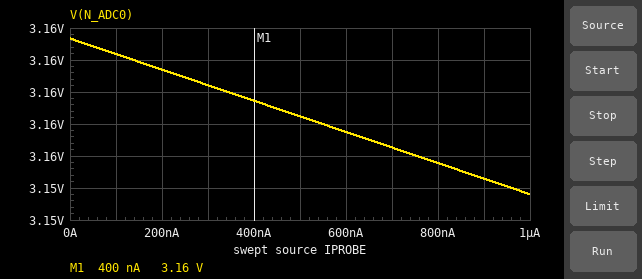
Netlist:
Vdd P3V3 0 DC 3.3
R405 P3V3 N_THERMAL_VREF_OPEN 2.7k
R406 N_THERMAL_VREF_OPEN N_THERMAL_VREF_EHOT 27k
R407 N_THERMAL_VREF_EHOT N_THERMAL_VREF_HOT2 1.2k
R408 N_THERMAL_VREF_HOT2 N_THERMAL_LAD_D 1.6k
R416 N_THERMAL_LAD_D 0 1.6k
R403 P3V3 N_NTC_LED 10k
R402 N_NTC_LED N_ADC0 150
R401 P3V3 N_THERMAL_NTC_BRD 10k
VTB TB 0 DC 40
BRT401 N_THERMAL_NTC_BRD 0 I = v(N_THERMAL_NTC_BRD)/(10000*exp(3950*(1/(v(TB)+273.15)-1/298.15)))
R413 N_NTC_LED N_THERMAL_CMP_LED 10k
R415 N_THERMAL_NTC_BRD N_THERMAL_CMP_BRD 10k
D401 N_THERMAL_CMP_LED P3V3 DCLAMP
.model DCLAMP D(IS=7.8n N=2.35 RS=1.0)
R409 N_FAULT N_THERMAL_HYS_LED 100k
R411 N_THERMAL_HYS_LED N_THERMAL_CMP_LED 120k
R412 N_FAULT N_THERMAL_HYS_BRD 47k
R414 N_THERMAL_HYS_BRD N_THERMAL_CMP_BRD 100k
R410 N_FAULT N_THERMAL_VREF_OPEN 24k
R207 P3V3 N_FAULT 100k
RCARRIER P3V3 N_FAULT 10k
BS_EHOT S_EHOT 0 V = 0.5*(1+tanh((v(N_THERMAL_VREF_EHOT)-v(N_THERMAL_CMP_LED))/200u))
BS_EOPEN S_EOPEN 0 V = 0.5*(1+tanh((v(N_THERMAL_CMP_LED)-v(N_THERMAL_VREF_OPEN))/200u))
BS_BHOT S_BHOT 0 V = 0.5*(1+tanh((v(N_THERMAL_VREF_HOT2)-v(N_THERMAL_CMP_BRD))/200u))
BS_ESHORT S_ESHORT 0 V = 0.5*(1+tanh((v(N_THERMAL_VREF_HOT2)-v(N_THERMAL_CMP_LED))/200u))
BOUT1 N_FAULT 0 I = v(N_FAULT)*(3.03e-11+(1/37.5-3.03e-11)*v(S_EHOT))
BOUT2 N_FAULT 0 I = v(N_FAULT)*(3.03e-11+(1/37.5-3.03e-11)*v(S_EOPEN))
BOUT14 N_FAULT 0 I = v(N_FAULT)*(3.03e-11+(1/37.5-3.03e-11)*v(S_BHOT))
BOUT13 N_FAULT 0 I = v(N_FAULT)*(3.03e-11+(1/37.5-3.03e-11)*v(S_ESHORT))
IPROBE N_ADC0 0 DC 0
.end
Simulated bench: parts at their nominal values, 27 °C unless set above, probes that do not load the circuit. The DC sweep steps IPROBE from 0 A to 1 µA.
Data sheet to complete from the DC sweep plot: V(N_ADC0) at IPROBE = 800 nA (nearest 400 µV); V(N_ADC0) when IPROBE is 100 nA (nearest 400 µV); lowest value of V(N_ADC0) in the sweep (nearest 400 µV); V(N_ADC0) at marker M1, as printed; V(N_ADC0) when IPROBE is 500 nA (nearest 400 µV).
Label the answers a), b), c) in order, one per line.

a) 3.1556 V
b) 3.1624 V
c) 3.1536 V
d) 3.16 V
e) 3.1584 V
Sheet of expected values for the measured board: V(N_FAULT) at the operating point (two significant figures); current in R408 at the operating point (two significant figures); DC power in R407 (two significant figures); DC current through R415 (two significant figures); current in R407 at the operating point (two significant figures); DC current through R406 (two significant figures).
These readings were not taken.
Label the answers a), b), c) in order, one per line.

a) 19 mV
b) 88 µA
c) 9.2 µW
d) 7.0 µA
e) 88 µA
f) 88 µA
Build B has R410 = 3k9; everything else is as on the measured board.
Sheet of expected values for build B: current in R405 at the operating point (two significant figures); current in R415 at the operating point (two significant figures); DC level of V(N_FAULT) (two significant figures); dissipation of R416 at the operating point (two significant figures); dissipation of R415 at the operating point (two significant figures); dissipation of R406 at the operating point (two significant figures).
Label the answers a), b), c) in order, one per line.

a) 530 µA
b) 6.9 µA
c) 32 mV
d) 5.7 µW
e) 480 nW
f) 96 µW
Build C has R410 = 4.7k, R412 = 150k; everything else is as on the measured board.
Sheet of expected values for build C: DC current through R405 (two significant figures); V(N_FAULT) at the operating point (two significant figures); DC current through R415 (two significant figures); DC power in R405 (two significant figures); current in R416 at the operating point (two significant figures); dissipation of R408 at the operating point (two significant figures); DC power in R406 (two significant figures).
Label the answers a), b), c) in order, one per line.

a) 480 µA
b) 30 mV
c) 4.2 µA
d) 630 µW
e) 64 µA
f) 6.5 µW
g) 110 µW
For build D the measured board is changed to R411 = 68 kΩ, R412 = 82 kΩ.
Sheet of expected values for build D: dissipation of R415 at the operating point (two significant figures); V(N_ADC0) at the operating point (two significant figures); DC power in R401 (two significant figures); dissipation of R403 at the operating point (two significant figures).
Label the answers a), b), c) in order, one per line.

a) 330 nW
b) 3.1 V
c) 470 µW
d) 3.0 µW
